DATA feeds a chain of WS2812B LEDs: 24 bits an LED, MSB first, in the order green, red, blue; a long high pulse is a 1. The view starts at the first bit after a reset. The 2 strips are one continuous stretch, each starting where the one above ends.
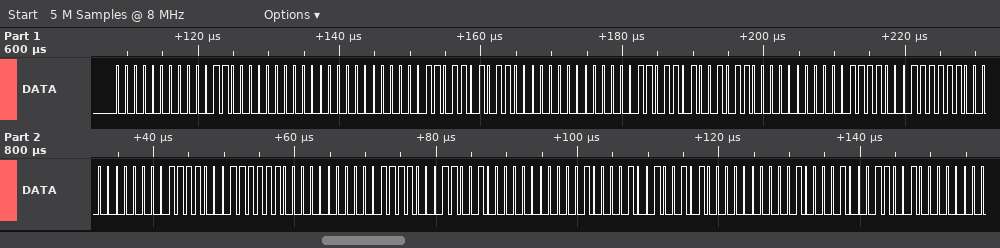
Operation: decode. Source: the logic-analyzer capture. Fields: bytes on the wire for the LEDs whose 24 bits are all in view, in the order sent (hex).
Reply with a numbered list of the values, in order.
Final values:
1. 00 18 00 00 1B 58 00 1B 4B 00 1E 3F 00 1E 3F 00 1E 32 00 21 25 00 21 19
